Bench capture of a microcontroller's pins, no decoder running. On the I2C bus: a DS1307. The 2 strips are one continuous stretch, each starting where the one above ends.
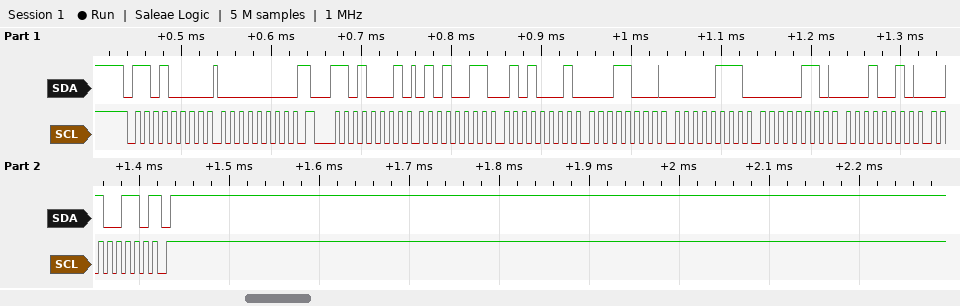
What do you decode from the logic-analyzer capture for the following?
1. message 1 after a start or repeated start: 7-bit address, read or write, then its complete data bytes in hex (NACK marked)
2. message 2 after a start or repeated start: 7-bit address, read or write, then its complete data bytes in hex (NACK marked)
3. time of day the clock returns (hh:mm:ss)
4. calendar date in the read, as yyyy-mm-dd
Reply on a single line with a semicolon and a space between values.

0x68 write: 00; 0x68 read: 53 51 18 07 06 12 26 NACK; 18:51:53; 2026-12-06
